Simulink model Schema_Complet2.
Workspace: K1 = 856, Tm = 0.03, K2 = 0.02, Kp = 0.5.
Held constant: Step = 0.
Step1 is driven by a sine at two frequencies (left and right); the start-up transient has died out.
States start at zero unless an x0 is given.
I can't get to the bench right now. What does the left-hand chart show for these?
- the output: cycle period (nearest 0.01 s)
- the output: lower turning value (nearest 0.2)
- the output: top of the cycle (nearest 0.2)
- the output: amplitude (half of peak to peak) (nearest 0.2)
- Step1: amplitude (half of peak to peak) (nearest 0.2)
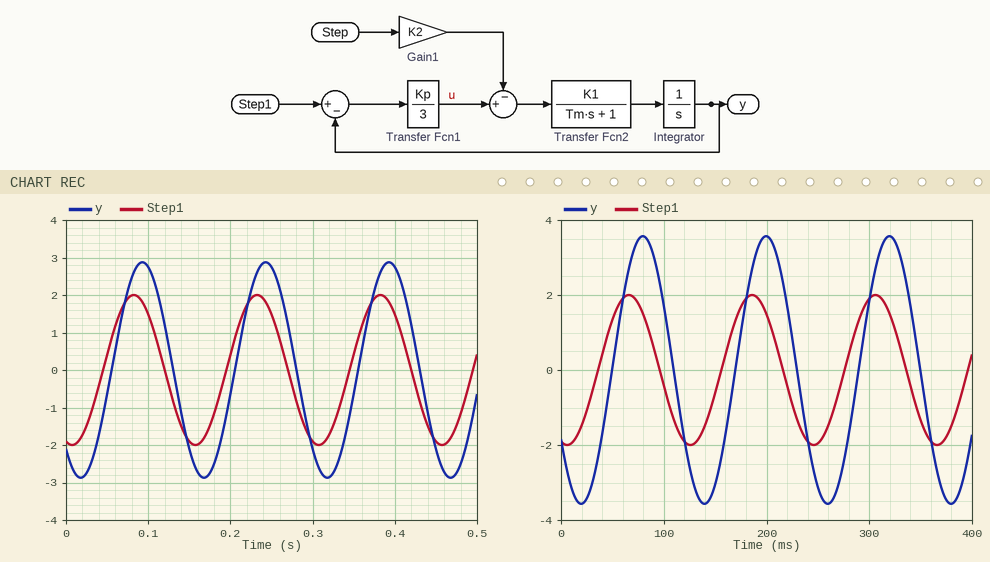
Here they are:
0.15 s
-2.8
2.8
2.8
2.0
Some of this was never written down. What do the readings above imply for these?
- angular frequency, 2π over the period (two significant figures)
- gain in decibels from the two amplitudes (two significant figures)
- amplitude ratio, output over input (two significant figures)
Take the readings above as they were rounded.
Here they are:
42 rad/s
2.9 dB
1.4
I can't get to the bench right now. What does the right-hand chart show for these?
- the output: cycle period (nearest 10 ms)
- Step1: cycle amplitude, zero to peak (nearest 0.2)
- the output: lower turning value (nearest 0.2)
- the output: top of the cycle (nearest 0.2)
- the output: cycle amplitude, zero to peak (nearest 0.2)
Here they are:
120 ms
2.0
-3.6
3.6
3.6
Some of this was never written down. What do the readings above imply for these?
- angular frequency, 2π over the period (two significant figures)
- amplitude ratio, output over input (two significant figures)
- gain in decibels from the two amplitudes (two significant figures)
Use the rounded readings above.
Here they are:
0.052 rad/ms
1.8
5.1 dB
